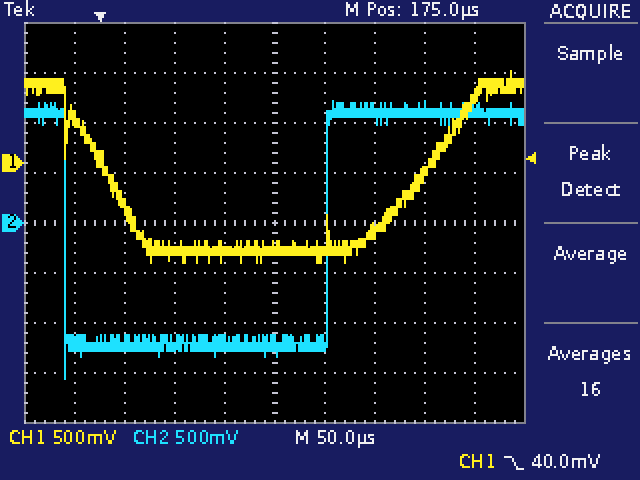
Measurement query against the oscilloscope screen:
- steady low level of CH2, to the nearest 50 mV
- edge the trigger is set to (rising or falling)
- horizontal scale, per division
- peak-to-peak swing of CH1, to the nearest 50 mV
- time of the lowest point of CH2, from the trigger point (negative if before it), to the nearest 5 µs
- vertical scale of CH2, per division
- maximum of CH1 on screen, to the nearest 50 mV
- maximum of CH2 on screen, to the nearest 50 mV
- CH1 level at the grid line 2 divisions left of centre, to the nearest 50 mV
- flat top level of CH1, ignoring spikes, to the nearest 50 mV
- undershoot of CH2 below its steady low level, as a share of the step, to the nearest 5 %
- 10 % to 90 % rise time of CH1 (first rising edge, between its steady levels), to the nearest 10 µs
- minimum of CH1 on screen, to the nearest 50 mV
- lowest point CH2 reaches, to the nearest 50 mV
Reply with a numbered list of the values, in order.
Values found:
1. -1.20 V
2. falling
3. 50 µs
4. 1.90 V
5. -35 µs
6. 500 mV
7. 900 mV
8. 1.20 V
9. -900 mV
10. 750 mV
11. 15 %
12. 100 µs
13. -1.00 V
14. -1.55 V
